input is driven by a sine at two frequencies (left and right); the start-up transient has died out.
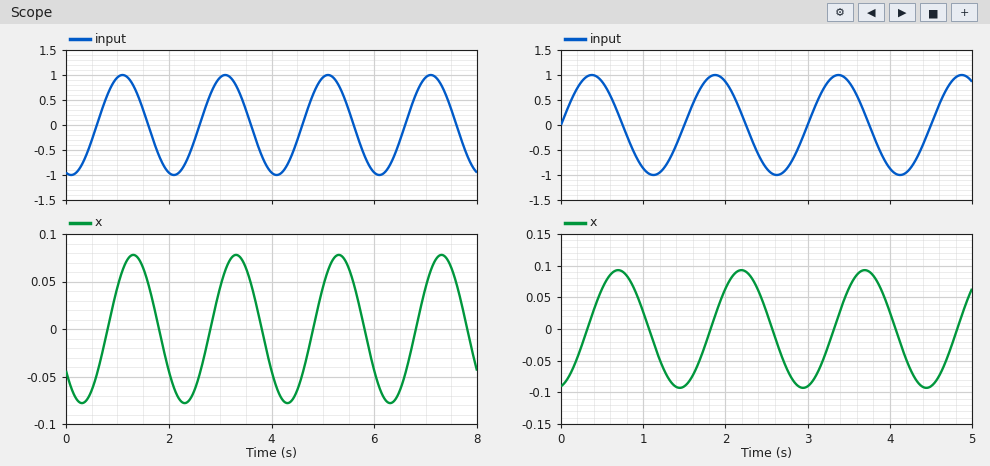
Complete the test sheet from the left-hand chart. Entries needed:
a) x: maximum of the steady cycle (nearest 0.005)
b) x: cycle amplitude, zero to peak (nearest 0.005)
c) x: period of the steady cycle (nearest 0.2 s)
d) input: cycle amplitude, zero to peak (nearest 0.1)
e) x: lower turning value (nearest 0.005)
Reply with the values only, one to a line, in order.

0.080
0.080
2.0 s
1.0
-0.080
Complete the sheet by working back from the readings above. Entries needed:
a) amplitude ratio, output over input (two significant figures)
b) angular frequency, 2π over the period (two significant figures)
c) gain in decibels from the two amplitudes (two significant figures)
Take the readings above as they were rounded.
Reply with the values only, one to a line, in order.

0.080
3.1 rad/s
-22 dB
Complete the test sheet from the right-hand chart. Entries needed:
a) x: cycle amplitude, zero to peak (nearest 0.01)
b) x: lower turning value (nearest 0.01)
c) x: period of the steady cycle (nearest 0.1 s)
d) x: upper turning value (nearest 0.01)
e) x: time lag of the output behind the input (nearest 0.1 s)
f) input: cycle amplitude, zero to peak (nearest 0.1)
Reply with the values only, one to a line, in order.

0.09
-0.09
1.5 s
0.09
0.3 s
1.0
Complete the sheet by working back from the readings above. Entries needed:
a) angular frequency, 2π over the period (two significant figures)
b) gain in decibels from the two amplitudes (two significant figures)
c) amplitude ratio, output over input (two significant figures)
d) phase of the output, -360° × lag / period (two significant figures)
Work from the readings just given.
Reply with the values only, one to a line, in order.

4.2 rad/s
-21 dB
0.090
-72°
